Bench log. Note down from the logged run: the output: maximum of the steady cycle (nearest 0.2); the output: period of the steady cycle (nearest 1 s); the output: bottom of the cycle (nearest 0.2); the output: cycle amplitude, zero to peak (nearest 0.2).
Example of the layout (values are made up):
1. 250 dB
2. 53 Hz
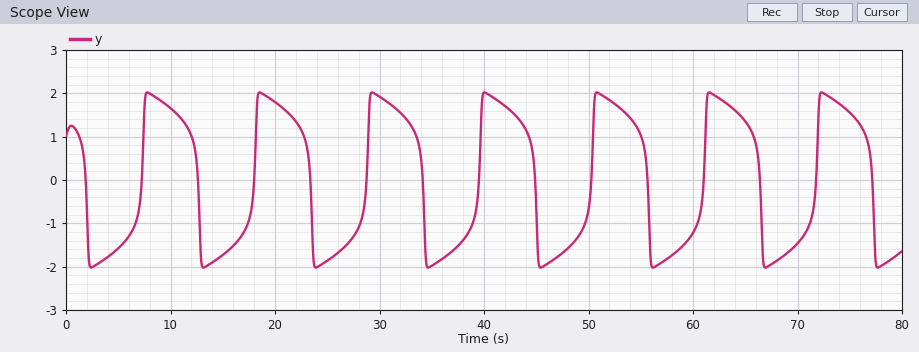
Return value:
1. 2.0
2. 11 s
3. -2.0
4. 2.0
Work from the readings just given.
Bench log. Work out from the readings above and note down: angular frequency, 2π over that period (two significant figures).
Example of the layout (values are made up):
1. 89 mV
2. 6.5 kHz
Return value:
1. 0.57 rad/s
